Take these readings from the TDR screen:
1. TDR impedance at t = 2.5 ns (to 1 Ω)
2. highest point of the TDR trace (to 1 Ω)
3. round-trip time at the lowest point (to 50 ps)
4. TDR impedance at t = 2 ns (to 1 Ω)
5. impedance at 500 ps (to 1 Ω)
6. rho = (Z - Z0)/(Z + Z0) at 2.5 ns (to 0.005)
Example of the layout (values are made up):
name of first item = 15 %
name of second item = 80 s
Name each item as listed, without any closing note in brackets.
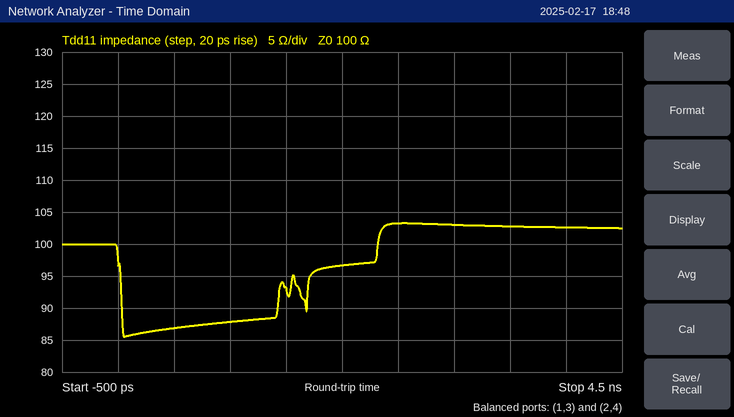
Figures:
TDR impedance at t = 2.5 ns = 103 Ω
highest point of the TDR trace = 103 Ω
round-trip time at the lowest point = 50 ps
TDR impedance at t = 2 ns = 97 Ω
impedance at 500 ps = 87 Ω
rho = (Z - Z0)/(Z + Z0) at 2.5 ns = +0.015
